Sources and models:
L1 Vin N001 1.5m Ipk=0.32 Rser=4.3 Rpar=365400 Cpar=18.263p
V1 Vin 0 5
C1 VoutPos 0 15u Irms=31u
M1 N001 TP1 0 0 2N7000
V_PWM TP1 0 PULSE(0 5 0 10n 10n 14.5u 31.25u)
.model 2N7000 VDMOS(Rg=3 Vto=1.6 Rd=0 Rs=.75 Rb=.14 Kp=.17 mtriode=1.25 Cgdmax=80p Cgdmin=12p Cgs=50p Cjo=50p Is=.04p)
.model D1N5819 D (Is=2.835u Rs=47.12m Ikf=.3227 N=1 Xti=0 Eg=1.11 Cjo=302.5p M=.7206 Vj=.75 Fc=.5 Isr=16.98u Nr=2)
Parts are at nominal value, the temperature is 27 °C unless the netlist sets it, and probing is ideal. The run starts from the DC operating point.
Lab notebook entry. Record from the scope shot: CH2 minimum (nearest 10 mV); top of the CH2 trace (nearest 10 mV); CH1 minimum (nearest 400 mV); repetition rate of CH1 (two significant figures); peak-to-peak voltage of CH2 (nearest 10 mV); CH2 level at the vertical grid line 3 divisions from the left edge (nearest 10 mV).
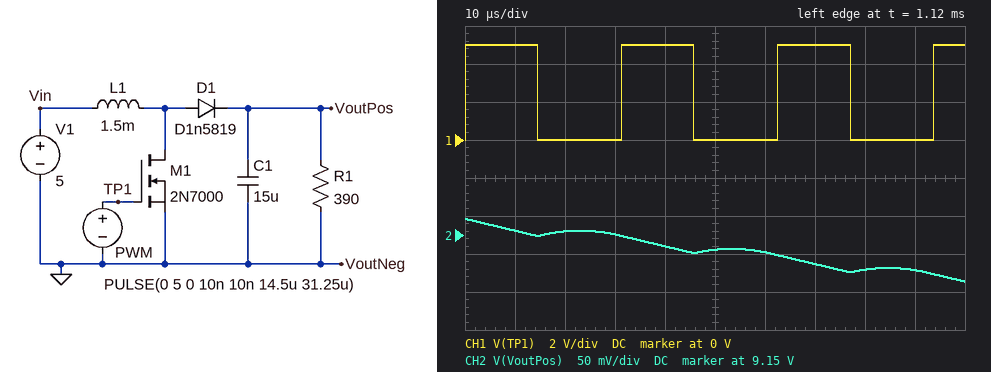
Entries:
9.09 V
9.17 V
0 V
32 kHz
80 mV
9.15 V
